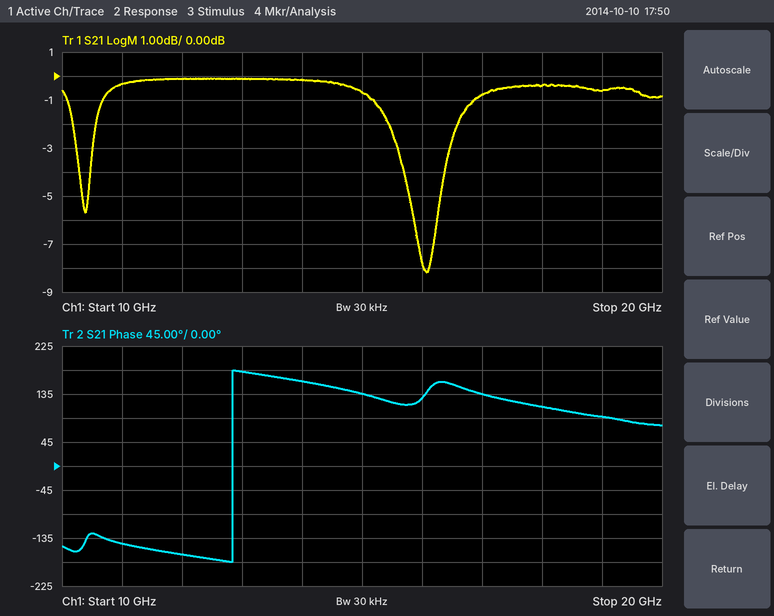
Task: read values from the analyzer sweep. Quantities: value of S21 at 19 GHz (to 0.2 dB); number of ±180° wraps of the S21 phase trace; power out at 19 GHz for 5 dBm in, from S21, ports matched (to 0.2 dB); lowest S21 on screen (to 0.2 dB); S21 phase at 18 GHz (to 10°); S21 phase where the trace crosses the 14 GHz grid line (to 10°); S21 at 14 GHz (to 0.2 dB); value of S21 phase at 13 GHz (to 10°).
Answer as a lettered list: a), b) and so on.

a) -0.6 dB
b) 1
c) 4.4 dBm
d) -8.2 dB
e) 110°
f) 160°
g) -0.2 dB
h) 180°
